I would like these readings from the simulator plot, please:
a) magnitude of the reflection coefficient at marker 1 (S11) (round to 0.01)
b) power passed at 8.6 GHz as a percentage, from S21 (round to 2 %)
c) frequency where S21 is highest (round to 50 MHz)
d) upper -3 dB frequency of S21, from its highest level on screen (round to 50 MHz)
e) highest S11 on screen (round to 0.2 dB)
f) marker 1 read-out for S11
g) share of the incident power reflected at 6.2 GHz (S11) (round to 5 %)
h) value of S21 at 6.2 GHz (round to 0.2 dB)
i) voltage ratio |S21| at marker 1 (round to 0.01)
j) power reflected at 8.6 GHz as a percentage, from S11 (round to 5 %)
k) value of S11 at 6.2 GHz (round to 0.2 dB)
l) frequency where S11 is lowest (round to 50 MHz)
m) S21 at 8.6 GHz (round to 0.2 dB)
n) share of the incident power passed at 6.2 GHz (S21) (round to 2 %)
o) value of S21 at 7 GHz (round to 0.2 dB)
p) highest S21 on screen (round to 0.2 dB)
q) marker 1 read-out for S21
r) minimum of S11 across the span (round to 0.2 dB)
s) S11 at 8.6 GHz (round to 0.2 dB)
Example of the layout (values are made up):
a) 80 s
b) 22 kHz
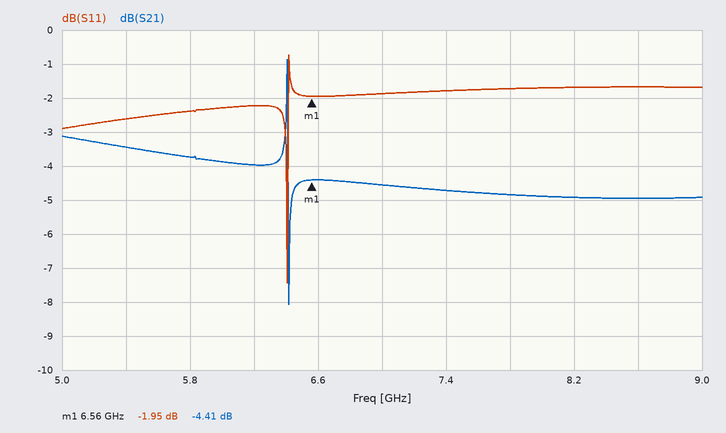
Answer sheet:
a) 0.80
b) 32 %
c) 6.40 GHz
d) 6.40 GHz
e) -0.8 dB
f) -1.95 dB
g) 60 %
h) -4.0 dB
i) 0.60
j) 70 %
k) -2.2 dB
l) 6.40 GHz
m) -5.0 dB
n) 40 %
o) -4.6 dB
p) -0.8 dB
q) -4.41 dB
r) -7.4 dB
s) -1.6 dB
